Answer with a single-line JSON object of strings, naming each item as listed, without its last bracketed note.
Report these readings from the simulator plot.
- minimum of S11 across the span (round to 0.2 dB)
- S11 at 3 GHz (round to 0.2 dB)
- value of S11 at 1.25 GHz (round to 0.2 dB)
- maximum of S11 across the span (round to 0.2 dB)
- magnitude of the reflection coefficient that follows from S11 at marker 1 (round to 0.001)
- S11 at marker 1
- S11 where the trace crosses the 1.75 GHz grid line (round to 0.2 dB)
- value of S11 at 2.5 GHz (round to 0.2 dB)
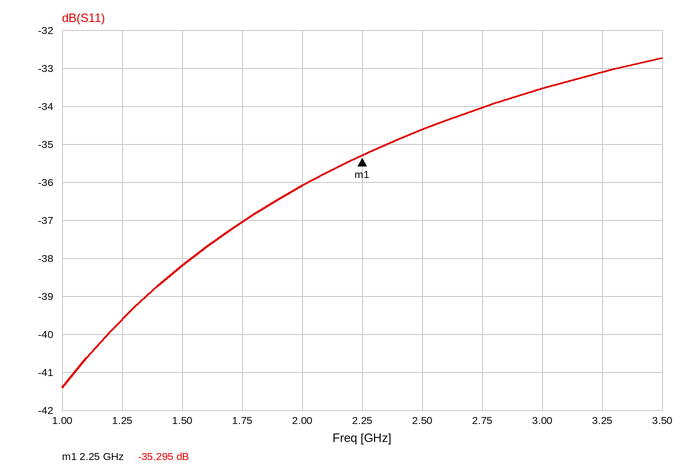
{"minimum of S11 across the span": "-41.4 dB", "S11 at 3 GHz": "-33.6 dB", "value of S11 at 1.25 GHz": "-39.6 dB", "maximum of S11 across the span": "-32.8 dB", "magnitude of the reflection coefficient that follows from S11 at marker 1": "0.017", "S11 at marker 1": "-35.295 dB", "S11 where the trace crosses the 1.75 GHz grid line": "-37.0 dB", "value of S11 at 2.5 GHz": "-34.6 dB"}
